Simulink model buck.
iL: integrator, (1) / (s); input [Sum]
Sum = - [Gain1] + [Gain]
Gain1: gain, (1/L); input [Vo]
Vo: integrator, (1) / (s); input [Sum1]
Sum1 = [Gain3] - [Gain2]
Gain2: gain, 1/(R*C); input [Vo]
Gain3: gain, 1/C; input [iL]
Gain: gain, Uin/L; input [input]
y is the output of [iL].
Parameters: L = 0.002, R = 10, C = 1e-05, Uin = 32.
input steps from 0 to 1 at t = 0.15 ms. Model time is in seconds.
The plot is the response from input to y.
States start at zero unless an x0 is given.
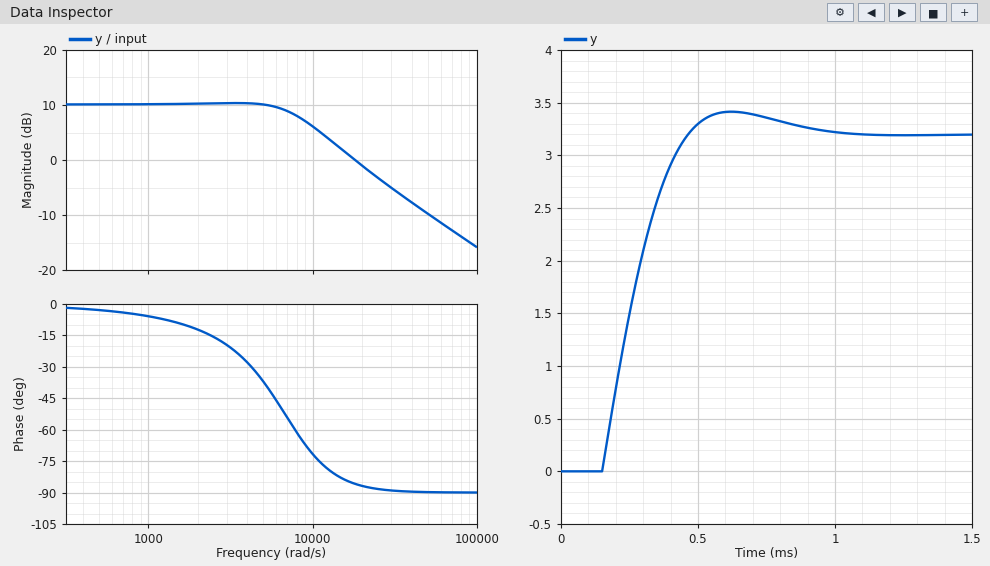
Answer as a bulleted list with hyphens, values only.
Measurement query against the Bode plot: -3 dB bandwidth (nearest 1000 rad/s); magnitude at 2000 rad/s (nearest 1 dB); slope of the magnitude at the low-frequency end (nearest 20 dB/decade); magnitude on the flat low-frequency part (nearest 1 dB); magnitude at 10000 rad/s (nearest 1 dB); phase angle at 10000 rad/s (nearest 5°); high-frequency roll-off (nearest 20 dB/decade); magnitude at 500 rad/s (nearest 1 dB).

- 9000 rad/s
- 10 dB
- 0 dB/decade
- 10 dB
- 6 dB
- -70°
- -20 dB/decade
- 10 dB
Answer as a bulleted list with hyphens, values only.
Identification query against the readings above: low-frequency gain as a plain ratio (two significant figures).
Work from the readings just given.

- 3.2
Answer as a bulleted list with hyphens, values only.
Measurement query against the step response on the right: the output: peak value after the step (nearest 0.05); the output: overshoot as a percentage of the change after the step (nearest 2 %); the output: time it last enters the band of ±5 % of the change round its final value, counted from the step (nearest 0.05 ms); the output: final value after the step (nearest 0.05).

- 3.40
- 6 %
- 0.60 ms
- 3.20
